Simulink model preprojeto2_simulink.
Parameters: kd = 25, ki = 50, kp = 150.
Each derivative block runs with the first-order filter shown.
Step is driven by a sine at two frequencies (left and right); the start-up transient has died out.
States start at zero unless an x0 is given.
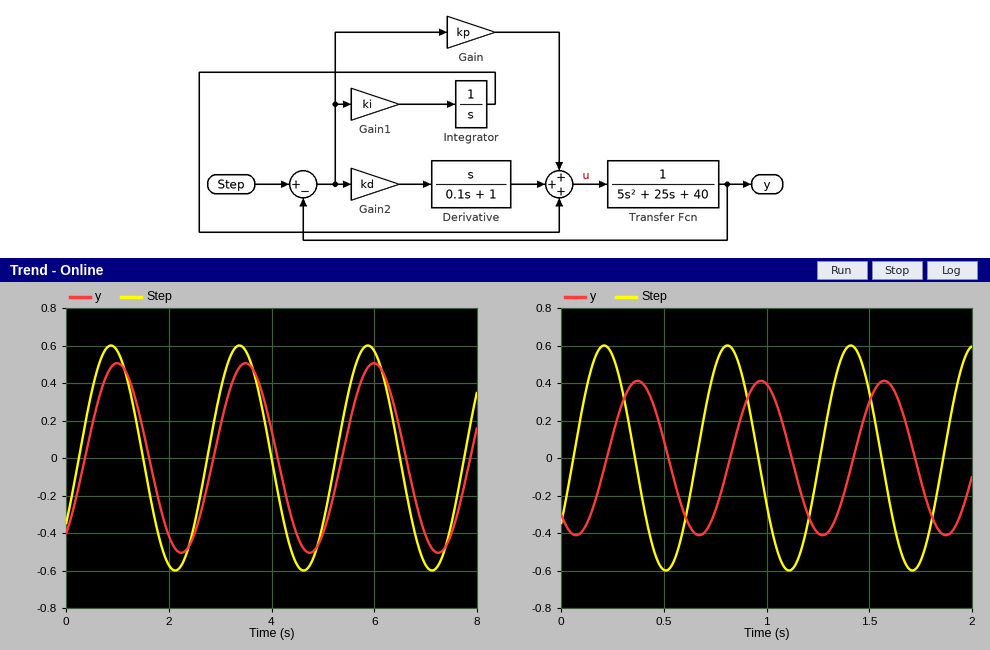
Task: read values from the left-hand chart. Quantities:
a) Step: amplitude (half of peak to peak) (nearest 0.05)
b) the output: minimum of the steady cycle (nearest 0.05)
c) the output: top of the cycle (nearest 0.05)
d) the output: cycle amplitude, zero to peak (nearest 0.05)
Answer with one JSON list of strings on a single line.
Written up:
["0.60", "-0.50", "0.50", "0.50"]
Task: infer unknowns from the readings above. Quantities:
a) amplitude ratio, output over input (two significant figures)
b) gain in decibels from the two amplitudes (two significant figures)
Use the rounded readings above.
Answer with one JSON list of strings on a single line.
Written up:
["0.83", "-1.6 dB"]
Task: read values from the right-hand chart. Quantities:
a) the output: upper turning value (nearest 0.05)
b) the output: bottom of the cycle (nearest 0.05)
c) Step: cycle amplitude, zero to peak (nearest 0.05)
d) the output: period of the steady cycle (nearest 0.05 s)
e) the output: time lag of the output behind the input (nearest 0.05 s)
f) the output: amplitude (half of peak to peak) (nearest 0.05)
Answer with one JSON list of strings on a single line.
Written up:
["0.40", "-0.40", "0.60", "0.60 s", "0.15 s", "0.40"]
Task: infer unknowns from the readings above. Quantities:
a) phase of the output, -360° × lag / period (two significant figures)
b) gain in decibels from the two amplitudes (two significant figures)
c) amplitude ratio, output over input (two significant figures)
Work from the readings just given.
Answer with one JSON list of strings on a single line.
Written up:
["-90°", "-3.5 dB", "0.67"]
